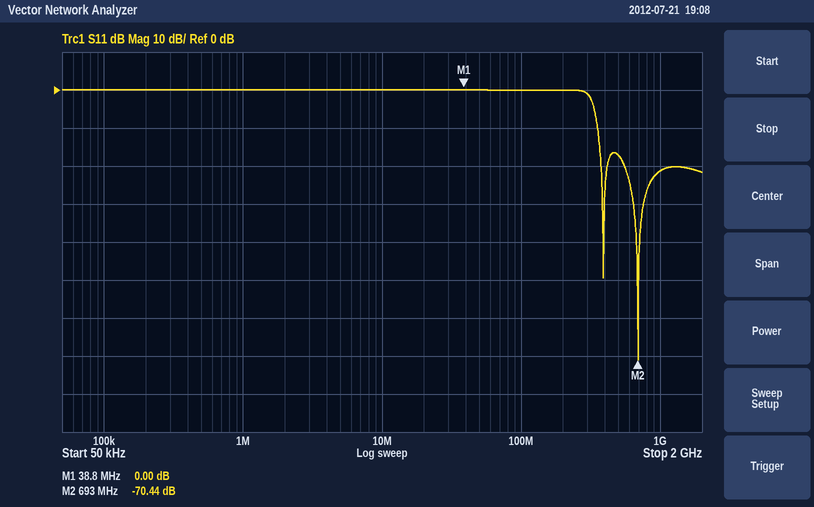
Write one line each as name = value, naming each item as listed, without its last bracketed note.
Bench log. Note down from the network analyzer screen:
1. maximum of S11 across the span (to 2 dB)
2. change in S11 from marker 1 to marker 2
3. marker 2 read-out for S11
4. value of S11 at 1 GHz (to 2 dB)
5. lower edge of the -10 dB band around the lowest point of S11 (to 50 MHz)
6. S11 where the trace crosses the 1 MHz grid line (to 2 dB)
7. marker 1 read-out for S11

maximum of S11 across the span = 0 dB
change in S11 from marker 1 to marker 2 = -70.44 dB
marker 2 read-out for S11 = -70.44 dB
value of S11 at 1 GHz = -22 dB
lower edge of the -10 dB band around the lowest point of S11 = 350 MHz
S11 where the trace crosses the 1 MHz grid line = 0 dB
marker 1 read-out for S11 = 0.00 dB
